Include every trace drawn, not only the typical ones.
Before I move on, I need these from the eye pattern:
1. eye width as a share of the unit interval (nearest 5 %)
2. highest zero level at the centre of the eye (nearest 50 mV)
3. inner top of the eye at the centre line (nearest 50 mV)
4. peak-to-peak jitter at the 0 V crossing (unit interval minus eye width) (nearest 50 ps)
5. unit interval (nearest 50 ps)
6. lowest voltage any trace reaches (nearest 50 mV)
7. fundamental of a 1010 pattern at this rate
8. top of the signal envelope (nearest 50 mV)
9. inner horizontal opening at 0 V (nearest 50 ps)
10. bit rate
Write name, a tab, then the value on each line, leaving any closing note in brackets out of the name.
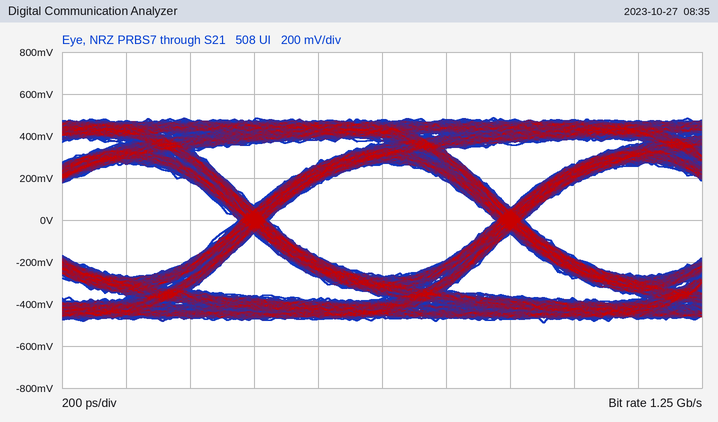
eye width as a share of the unit interval	90 %
highest zero level at the centre of the eye	-250 mV
inner top of the eye at the centre line	250 mV
peak-to-peak jitter at the 0 V crossing (unit interval minus eye width)	100 ps
unit interval	800 ps
lowest voltage any trace reaches	-500 mV
fundamental of a 1010 pattern at this rate	625 MHz
top of the signal envelope	500 mV
inner horizontal opening at 0 V	700 ps
bit rate	1.25 Gb/s
